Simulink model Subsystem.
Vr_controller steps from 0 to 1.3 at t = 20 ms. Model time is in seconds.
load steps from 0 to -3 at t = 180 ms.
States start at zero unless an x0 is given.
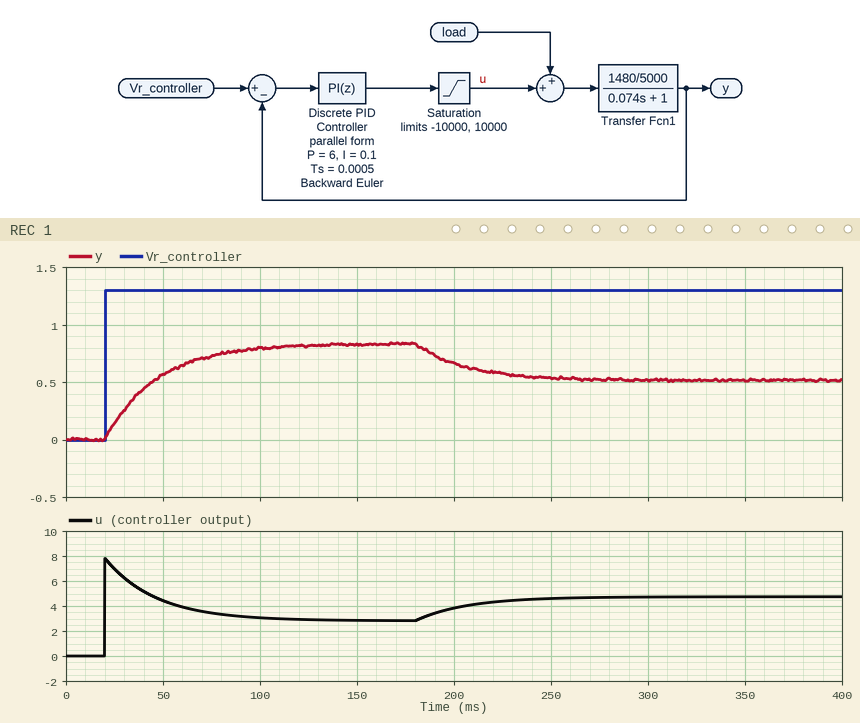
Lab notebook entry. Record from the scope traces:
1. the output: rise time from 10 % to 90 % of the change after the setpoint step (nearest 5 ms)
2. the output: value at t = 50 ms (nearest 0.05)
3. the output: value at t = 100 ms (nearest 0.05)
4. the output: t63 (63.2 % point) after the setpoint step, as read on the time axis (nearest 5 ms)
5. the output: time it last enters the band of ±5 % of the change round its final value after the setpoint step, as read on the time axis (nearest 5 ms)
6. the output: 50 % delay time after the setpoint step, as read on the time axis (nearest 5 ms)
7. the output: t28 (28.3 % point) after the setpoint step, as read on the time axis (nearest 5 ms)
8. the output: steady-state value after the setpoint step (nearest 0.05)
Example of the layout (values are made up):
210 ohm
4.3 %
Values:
60 ms
0.55
0.80
45 ms
105 ms
40 ms
30 ms
0.85
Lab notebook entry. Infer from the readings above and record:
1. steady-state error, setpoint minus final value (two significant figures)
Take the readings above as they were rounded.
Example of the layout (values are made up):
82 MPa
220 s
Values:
0.45
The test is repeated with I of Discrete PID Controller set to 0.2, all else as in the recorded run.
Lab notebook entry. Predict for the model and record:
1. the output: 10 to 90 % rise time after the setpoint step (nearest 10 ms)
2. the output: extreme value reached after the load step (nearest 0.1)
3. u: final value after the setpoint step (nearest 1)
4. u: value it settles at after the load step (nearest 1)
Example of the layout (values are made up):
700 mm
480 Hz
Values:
60 ms
0.5
3
5
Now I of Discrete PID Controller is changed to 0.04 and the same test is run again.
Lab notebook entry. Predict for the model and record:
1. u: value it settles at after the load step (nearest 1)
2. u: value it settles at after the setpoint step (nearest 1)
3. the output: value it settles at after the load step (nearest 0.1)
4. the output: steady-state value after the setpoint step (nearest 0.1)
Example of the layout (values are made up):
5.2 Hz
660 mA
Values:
5
3
0.5
0.8
